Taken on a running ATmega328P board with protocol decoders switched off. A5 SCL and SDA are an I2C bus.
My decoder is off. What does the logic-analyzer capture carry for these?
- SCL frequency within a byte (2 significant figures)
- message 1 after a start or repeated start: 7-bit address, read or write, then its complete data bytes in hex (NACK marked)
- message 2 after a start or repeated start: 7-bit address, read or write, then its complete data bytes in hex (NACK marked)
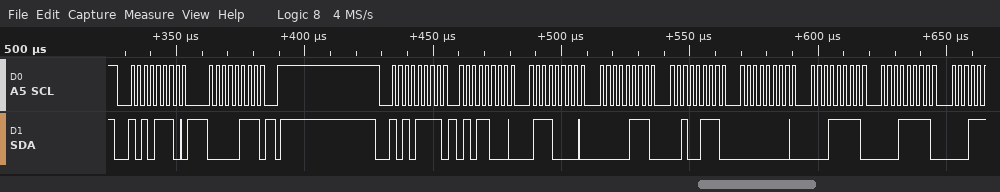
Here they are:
400 kHz
0x57 write: 07
0x57 read: 58 70 07 27 00 1F 1F
